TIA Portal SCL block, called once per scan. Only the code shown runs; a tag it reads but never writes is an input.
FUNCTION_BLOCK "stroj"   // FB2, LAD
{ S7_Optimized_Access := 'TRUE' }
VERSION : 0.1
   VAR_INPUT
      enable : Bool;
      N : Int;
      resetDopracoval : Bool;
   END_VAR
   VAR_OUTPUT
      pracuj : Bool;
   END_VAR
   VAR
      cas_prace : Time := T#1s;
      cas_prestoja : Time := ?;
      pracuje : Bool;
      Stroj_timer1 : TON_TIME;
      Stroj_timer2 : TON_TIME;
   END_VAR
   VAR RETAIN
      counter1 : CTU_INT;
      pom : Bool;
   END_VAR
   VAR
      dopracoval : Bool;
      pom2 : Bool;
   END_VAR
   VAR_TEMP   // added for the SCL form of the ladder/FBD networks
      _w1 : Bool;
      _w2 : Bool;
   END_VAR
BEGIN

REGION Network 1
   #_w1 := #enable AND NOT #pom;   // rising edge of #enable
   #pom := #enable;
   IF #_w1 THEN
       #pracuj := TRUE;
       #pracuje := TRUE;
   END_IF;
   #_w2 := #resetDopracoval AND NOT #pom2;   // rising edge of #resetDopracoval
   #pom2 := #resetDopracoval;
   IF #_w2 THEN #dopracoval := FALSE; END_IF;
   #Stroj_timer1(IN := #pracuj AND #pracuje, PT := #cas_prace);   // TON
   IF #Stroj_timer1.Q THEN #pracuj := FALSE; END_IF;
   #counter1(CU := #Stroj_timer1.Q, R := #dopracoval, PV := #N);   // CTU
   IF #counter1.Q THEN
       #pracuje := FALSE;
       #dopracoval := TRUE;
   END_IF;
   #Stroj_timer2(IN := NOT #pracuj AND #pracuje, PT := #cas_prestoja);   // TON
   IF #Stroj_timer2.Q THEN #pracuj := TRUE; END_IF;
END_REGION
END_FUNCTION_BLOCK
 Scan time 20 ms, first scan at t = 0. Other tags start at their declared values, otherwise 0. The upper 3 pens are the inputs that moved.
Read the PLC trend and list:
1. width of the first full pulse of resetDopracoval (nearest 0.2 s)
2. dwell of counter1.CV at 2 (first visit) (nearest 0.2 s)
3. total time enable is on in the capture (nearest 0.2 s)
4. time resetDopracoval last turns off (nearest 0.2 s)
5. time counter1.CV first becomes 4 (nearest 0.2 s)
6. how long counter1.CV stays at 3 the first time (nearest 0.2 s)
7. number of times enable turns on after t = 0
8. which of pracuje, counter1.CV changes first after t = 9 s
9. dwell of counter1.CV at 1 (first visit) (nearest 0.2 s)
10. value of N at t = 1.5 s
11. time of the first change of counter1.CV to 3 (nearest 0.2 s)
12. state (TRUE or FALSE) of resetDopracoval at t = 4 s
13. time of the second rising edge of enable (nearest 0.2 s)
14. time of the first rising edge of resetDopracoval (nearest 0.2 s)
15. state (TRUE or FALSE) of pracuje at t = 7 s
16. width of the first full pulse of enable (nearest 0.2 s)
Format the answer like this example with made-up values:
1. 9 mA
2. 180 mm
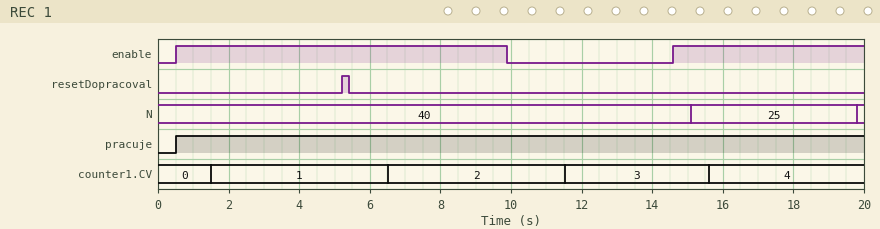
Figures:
1. 0.2 s
2. 5.0 s
3. 14.8 s
4. 5.4 s
5. 15.6 s
6. 4.0 s
7. 2
8. counter1.CV
9. 5.0 s
10. 40
11. 11.6 s
12. FALSE
13. 14.6 s
14. 5.2 s
15. TRUE
16. 9.4 s
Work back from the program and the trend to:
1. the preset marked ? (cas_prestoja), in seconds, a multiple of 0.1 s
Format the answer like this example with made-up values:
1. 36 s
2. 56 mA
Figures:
1. 4.0 s
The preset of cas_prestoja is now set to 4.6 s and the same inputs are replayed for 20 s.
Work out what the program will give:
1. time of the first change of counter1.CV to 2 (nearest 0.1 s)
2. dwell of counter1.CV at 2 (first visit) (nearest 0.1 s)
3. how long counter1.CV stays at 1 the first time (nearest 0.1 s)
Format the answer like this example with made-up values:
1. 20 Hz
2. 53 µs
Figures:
1. 7.1 s
2. 5.6 s
3. 5.6 s
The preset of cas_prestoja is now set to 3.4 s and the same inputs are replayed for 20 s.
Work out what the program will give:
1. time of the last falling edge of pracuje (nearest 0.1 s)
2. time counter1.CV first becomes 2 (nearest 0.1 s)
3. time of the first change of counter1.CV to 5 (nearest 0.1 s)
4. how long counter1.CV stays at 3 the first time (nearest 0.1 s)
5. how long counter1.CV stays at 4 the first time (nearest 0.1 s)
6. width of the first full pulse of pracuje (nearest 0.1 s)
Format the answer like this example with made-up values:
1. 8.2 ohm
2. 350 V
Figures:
1. 19.8 s
2. 5.9 s
3. 19.2 s
4. 4.4 s
5. 4.4 s
6. 19.3 s
